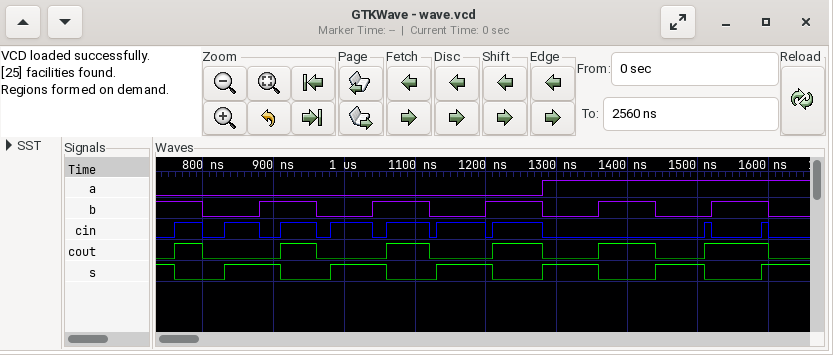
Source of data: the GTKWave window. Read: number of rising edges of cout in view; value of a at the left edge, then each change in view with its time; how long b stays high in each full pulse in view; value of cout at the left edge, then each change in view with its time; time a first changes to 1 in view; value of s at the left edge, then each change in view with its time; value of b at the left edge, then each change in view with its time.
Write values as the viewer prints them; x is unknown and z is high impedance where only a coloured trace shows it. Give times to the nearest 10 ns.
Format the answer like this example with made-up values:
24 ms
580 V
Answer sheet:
6
0, 1 at 1280 ns
80 ns, 80 ns, 80 ns, 80 ns, 80 ns
0, 1 at 760 ns, 0 at 800 ns, 1 at 910 ns, 0 at 960 ns, 1 at 1060 ns, 0 at 1120 ns, 1 at 1210 ns, 0 at 1280 ns, 1 at 1360 ns, 0 at 1440 ns, 1 at 1510 ns, 0 at 1600 ns
1280 ns
1, 0 at 760 ns, 1 at 830 ns, 0 at 910 ns, 1 at 980 ns, 0 at 1060 ns, 1 at 1130 ns, 0 at 1210 ns, 1 at 1280 ns, 0 at 1360 ns, 1 at 1440 ns, 0 at 1510 ns, 1 at 1590 ns
1, 0 at 800 ns, 1 at 880 ns, 0 at 960 ns, 1 at 1040 ns, 0 at 1120 ns, 1 at 1200 ns, 0 at 1280 ns, 1 at 1360 ns, 0 at 1440 ns, 1 at 1520 ns, 0 at 1600 ns
